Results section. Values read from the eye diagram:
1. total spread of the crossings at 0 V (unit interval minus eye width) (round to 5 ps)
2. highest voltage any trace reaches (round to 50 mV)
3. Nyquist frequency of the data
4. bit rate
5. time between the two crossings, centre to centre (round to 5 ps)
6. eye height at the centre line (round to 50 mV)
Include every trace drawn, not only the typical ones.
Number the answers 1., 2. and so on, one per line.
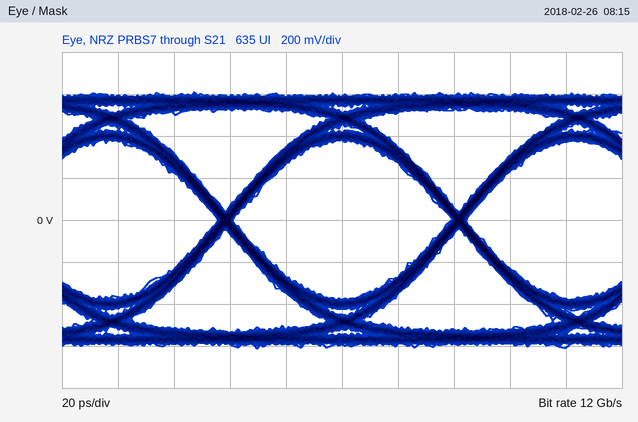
1. 5 ps
2. 600 mV
3. 6 GHz
4. 12 Gb/s
5. 85 ps
6. 750 mV
